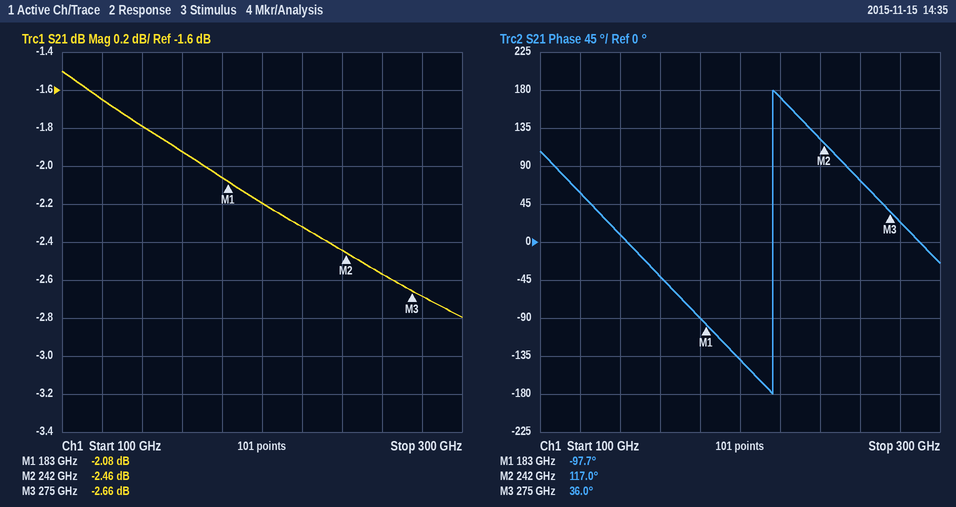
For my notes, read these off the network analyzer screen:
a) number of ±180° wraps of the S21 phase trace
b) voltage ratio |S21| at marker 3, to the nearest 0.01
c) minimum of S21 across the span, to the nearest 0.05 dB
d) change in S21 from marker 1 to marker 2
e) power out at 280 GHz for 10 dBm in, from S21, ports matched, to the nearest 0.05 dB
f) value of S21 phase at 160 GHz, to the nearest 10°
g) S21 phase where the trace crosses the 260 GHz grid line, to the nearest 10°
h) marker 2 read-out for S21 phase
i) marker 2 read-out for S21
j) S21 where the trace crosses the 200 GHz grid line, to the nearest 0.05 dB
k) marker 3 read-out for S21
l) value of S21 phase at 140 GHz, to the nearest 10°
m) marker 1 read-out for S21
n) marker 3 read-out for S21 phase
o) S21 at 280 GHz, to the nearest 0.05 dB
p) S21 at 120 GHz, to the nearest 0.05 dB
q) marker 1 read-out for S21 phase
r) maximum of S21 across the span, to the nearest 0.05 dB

1
0.74
-2.80 dB
-0.38 dB
7.30 dBm
-40°
70°
117.0°
-2.46 dB
-2.20 dB
-2.66 dB
10°
-2.08 dB
36.0°
-2.70 dB
-1.65 dB
-97.7°
-1.50 dB
